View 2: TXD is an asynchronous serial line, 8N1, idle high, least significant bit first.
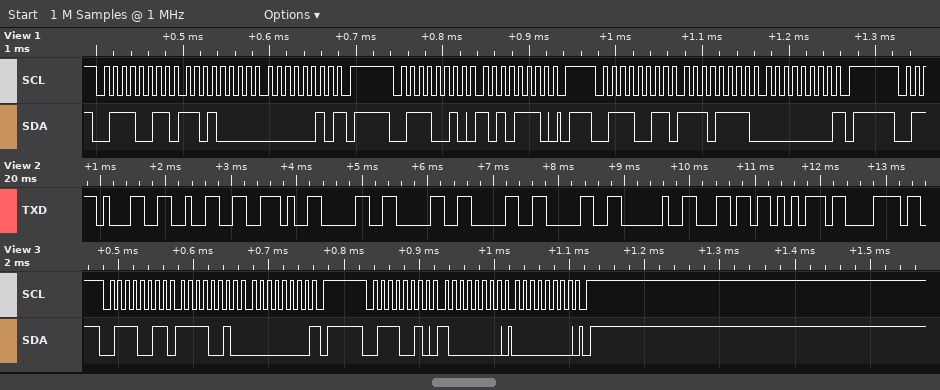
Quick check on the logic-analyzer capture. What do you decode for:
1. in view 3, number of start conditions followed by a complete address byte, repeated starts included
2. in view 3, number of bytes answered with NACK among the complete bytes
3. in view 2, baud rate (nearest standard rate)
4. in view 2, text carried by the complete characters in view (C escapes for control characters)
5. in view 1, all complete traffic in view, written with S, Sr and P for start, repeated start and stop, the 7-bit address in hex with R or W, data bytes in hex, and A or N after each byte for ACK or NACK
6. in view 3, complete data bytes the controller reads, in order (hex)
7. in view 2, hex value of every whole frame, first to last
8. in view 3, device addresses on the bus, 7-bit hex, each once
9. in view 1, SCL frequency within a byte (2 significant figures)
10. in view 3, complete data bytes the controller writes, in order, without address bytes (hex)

2
1
9600 baud
"12.0000 lux"
S 39R A D0 A 02 N P S 39W A AE A P S 39R A EF A 00 N P
F2 00
31 32 2E 30 30 30 30 20 6C 75 78
0x39
100 kHz
80 00
